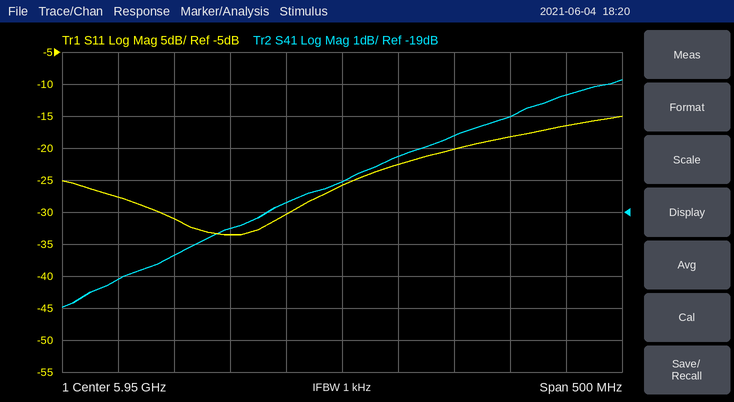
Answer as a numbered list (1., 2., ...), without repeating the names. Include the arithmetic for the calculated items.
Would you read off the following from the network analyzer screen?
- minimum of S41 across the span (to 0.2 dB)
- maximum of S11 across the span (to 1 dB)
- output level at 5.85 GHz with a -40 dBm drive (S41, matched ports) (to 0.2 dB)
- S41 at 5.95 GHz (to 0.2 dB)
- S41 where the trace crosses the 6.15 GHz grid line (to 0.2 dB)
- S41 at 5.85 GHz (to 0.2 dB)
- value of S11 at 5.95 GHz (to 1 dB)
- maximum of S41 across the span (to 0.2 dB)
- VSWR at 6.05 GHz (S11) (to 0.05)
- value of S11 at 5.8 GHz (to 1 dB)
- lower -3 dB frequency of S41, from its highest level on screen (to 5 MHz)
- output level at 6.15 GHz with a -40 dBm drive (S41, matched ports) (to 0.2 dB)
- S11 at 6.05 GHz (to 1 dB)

1. -22.0 dB
2. -15 dB
3. -40 dBm + (-19.6 dB) = -59.6 dBm
4. -18.0 dB
5. -15.4 dB
6. -19.6 dB
7. -26 dB
8. -14.8 dB
9. |Γ| = 10^(-20/20) = 0.1000; VSWR = (1 + 0.1000)/(1 − 0.1000) ≈ 1.22, so 1.20 to the nearest 0.05
10. -31 dB
11. 5.960 GHz
12. -40 dBm + (-15.4 dB) = -55.4 dBm
13. -20 dB
